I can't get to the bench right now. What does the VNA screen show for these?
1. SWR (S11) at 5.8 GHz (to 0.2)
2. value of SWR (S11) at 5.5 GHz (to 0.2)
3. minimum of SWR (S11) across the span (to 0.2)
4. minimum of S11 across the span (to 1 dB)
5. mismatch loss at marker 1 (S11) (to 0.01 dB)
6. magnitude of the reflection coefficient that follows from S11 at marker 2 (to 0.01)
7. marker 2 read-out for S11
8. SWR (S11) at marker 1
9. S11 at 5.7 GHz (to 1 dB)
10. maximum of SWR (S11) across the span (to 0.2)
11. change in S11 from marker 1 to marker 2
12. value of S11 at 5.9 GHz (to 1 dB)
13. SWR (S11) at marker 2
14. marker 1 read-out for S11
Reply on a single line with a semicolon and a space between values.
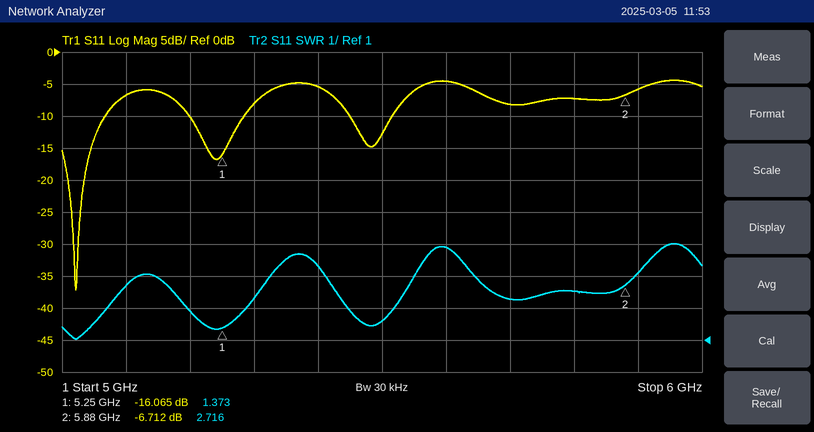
2.6; 1.6; 1.0; -37 dB; 0.11 dB; 0.46; -6.712 dB; 1.373; -8 dB; 4.0; 9.353 dB; -6 dB; 2.716; -16.065 dB
